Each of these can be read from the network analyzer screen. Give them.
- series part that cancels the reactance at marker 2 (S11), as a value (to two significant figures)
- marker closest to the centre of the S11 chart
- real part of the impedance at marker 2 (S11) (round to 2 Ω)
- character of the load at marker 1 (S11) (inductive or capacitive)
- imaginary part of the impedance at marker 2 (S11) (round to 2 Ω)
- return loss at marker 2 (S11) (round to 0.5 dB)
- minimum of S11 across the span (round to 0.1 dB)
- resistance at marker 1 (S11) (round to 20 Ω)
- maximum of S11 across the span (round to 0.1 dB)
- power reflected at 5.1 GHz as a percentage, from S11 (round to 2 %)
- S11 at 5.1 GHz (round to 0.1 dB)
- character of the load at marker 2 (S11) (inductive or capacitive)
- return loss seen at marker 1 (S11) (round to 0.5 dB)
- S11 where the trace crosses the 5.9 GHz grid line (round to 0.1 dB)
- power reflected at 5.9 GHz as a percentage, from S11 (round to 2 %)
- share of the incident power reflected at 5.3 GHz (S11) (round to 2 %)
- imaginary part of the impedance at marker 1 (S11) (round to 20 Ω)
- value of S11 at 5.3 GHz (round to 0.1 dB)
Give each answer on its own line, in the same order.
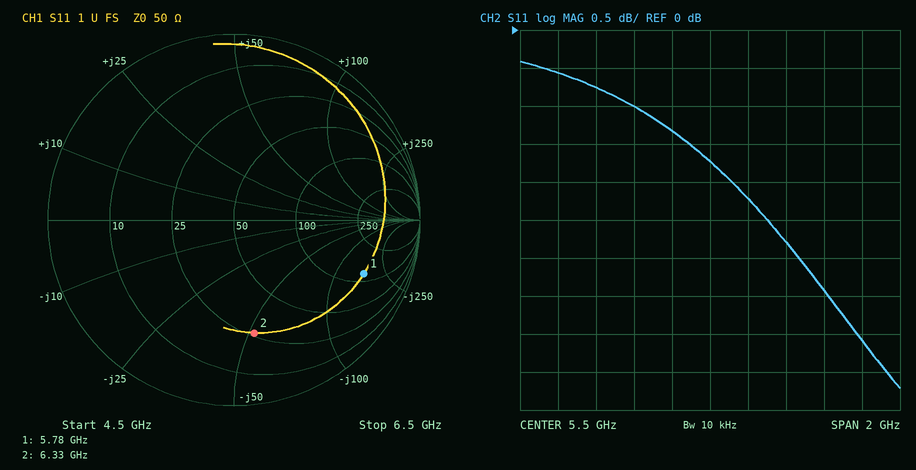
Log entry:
1.3 nH
marker 2
26 Ω
capacitive
-52 Ω
4.0 dB
-4.7 dB
120 Ω
-0.4 dB
80 %
-1.0 dB
capacitive
2.5 dB
-2.8 dB
52 %
74 %
-160 Ω
-1.3 dB
